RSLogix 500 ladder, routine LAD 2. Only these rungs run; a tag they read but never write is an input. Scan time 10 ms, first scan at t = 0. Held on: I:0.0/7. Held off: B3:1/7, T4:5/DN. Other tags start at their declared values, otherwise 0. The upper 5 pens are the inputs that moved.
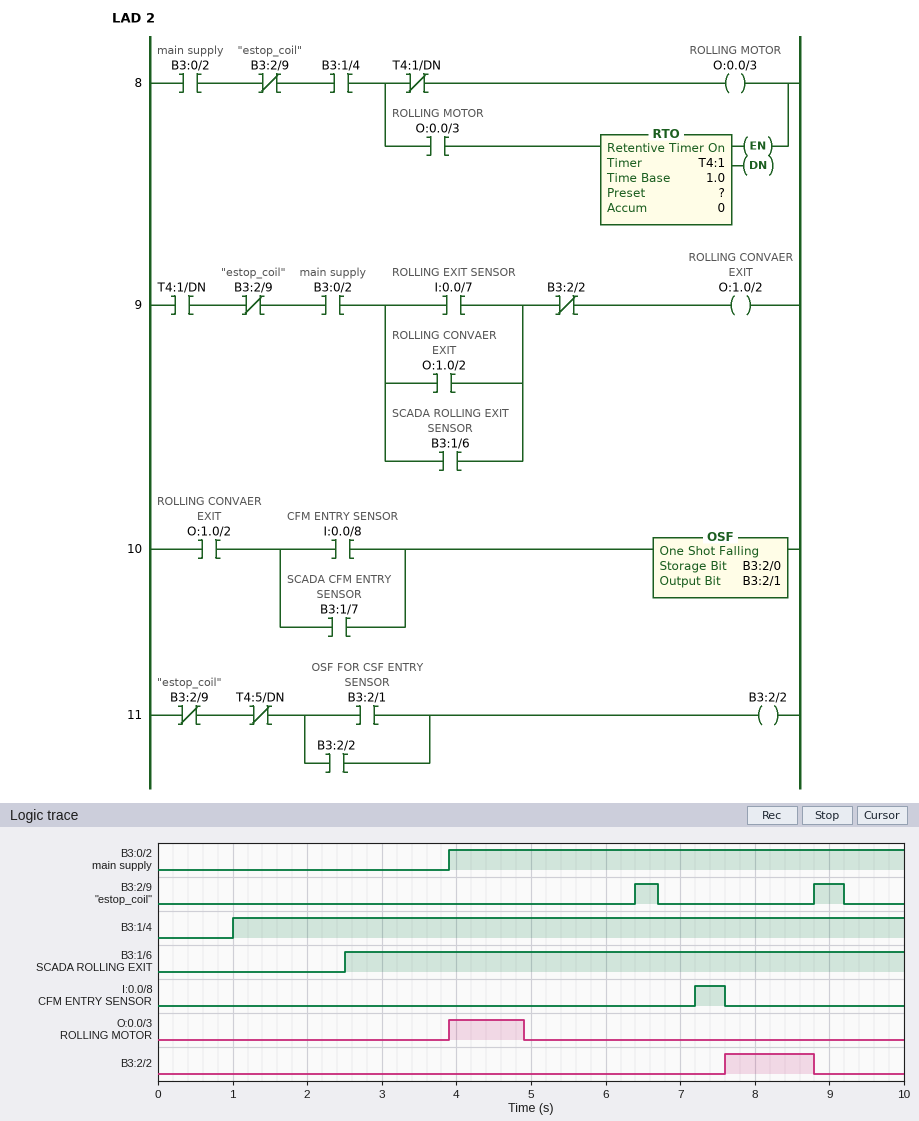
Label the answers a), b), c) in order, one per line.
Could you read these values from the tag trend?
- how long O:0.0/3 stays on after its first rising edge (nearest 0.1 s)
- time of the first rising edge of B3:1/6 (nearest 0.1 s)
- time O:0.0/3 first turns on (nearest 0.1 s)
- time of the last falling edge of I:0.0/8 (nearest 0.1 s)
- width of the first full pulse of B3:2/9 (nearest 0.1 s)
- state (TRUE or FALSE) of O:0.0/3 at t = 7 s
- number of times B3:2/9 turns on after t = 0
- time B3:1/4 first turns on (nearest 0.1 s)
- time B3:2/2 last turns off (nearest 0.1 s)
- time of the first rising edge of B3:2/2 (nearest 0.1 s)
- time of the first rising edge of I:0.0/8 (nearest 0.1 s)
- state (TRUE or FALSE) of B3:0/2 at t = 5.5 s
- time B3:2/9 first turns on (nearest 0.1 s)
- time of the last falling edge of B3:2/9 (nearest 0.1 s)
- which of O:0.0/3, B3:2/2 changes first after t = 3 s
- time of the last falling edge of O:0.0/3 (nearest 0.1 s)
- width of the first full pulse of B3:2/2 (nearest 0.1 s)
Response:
a) 1.0 s
b) 2.5 s
c) 3.9 s
d) 7.6 s
e) 0.3 s
f) FALSE
g) 2
h) 1.0 s
i) 8.8 s
j) 7.6 s
k) 7.2 s
l) TRUE
m) 6.4 s
n) 9.2 s
o) O:0.0/3
p) 4.9 s
q) 1.2 s
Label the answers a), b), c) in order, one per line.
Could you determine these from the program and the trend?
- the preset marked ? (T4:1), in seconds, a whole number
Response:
a) 1 s
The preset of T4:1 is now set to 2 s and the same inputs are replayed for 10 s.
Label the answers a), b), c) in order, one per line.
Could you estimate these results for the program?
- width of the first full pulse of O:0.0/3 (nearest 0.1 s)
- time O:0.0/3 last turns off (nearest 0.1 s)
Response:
a) 2.0 s
b) 5.9 s
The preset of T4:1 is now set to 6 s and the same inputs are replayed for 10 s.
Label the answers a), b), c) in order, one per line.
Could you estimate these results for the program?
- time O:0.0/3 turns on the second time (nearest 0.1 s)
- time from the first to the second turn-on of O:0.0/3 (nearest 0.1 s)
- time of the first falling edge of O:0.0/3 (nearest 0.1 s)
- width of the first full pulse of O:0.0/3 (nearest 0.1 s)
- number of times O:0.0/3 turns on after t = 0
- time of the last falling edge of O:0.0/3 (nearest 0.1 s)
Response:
a) 6.7 s
b) 2.8 s
c) 6.4 s
d) 2.5 s
e) 3
f) 8.8 s
